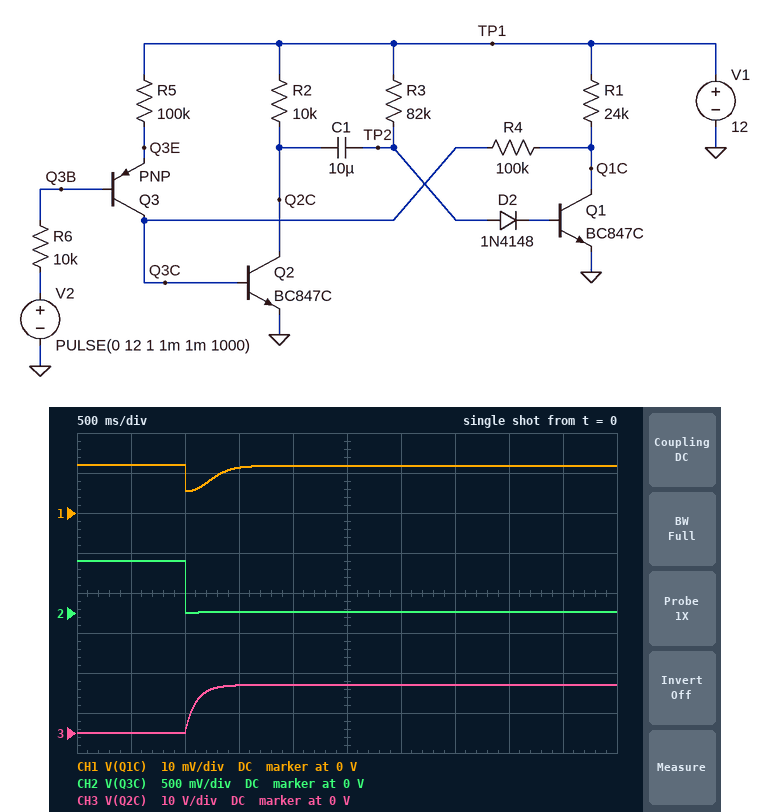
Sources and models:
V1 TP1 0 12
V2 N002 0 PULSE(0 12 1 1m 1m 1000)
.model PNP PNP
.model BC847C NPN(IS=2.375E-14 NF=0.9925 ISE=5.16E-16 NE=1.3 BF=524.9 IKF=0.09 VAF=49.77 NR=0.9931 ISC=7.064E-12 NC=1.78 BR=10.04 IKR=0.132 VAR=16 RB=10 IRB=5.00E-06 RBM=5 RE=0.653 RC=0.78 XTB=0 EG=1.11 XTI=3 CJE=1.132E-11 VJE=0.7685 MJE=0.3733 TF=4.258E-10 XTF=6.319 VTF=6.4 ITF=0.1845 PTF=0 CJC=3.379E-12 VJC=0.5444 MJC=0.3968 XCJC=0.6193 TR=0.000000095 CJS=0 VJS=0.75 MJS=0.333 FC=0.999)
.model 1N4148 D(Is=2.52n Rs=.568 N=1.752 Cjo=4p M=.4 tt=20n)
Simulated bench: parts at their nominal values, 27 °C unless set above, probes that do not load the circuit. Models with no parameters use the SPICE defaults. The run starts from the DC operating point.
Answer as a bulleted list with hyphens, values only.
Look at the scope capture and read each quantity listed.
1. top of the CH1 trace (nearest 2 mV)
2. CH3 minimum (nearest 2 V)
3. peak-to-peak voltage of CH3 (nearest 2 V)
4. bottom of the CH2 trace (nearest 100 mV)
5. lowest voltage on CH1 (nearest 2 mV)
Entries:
- 12 mV
- 0 V
- 12 V
- 0 V
- 6 mV
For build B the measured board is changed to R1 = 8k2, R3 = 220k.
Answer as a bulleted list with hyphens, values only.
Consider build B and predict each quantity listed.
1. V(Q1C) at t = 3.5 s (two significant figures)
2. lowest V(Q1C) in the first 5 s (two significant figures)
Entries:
- 42 mV
- 9.0 mV
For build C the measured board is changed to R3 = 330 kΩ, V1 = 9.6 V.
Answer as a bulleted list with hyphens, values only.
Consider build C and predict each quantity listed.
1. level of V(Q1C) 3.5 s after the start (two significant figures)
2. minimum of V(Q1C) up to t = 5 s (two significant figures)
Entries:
- 29 mV
- 5.0 mV
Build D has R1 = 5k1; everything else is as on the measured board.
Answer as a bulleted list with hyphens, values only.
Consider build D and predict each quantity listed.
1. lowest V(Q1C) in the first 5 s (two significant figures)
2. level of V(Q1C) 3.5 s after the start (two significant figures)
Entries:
- 12 mV
- 34 mV
